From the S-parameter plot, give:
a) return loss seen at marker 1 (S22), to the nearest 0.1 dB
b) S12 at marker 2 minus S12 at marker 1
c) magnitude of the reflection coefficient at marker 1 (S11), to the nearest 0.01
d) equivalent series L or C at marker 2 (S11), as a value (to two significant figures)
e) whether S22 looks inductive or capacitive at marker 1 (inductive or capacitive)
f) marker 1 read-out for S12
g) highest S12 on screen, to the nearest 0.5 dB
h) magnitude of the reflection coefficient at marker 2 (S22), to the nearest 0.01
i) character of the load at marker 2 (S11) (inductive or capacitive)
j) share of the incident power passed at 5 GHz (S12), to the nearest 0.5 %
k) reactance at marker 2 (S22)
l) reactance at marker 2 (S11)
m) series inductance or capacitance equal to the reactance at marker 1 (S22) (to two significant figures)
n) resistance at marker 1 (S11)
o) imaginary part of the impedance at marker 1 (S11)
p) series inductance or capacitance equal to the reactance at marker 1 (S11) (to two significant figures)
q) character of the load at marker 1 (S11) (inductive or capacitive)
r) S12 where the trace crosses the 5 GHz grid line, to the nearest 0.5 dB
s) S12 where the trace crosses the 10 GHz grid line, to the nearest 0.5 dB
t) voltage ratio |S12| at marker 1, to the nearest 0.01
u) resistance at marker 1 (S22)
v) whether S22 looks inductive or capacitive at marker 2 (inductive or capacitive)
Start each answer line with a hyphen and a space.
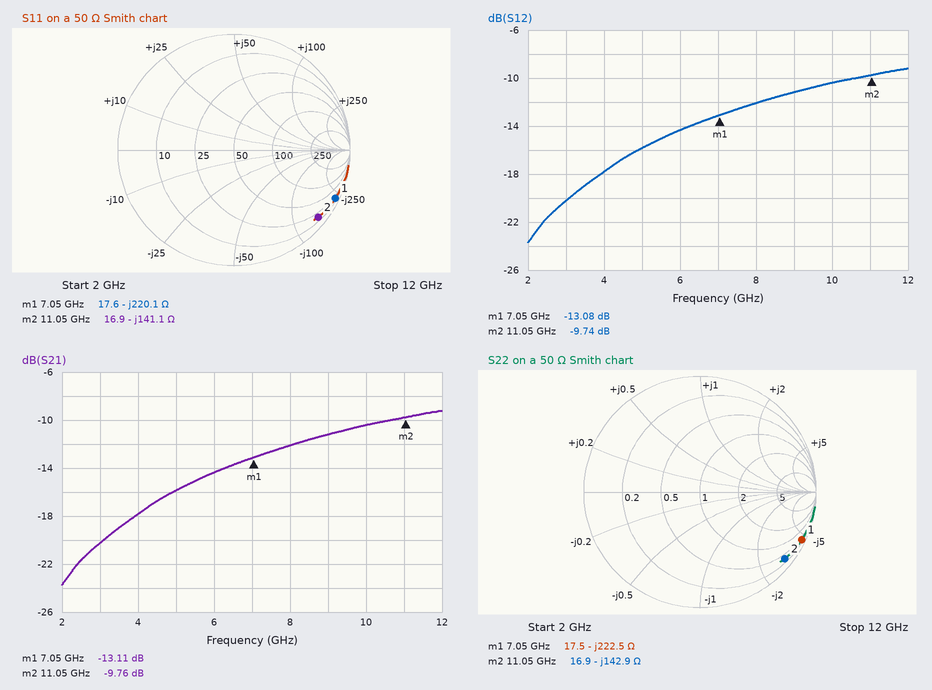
- 0.3 dB
- 3.34 dB
- 0.97
- 100 fF
- capacitive
- -13.08 dB
- -9.0 dB
- 0.93
- capacitive
- 2.5 %
- -142.9 Ω
- -141.1 Ω
- 100 fF
- 17.6 Ω
- -220.1 Ω
- 100 fF
- capacitive
- -16.0 dB
- -10.5 dB
- 0.22
- 17.5 Ω
- capacitive
